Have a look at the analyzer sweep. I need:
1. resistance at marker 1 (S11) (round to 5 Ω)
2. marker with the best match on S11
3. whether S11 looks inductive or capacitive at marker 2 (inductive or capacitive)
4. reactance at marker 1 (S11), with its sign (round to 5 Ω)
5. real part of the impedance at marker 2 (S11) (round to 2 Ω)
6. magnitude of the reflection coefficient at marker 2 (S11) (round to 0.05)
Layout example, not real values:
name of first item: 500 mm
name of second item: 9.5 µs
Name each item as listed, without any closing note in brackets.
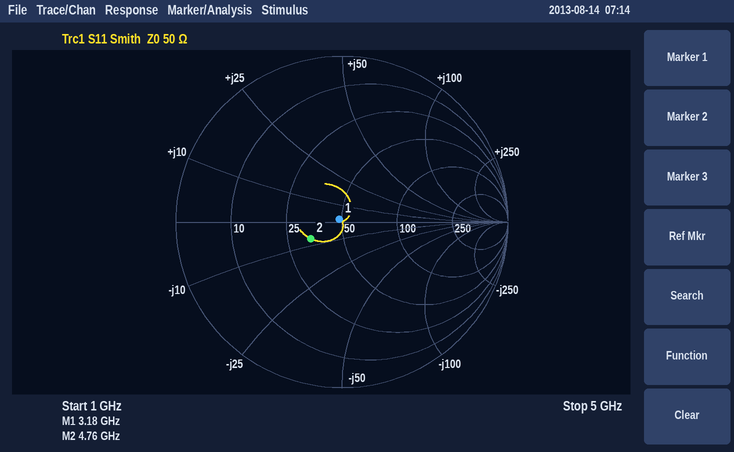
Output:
resistance at marker 1 (S11): 50 Ω
marker with the best match on S11: marker 1
whether S11 looks inductive or capacitive at marker 2: capacitive
reactance at marker 1 (S11), with its sign: 0 Ω
real part of the impedance at marker 2 (S11): 34 Ω
magnitude of the reflection coefficient at marker 2 (S11): 0.20
